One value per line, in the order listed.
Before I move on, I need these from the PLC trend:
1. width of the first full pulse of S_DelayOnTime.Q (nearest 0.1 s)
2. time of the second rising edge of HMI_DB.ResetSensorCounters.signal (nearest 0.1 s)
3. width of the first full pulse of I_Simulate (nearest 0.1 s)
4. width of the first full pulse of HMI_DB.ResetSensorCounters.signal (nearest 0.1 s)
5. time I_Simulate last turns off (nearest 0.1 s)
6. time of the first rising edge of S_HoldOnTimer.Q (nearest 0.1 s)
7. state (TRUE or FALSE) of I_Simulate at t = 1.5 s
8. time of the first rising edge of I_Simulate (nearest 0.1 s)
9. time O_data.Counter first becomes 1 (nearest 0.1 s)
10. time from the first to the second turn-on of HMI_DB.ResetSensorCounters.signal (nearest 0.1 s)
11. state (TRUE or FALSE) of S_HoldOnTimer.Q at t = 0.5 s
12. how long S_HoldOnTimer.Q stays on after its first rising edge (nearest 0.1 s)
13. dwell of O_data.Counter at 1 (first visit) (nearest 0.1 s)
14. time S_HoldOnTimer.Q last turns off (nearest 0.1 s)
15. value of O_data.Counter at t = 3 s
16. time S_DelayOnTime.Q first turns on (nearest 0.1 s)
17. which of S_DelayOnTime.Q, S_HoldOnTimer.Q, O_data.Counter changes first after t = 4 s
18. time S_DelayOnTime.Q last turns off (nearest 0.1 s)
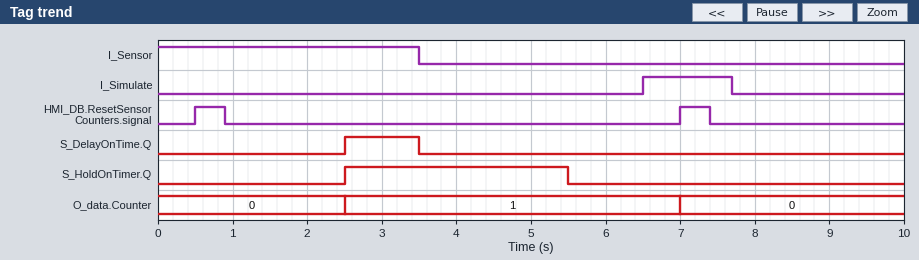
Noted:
1.0 s
7.0 s
1.2 s
0.4 s
7.7 s
2.5 s
FALSE
6.5 s
2.5 s
6.5 s
FALSE
3.0 s
4.5 s
5.5 s
1
2.5 s
S_HoldOnTimer.Q
3.5 s
